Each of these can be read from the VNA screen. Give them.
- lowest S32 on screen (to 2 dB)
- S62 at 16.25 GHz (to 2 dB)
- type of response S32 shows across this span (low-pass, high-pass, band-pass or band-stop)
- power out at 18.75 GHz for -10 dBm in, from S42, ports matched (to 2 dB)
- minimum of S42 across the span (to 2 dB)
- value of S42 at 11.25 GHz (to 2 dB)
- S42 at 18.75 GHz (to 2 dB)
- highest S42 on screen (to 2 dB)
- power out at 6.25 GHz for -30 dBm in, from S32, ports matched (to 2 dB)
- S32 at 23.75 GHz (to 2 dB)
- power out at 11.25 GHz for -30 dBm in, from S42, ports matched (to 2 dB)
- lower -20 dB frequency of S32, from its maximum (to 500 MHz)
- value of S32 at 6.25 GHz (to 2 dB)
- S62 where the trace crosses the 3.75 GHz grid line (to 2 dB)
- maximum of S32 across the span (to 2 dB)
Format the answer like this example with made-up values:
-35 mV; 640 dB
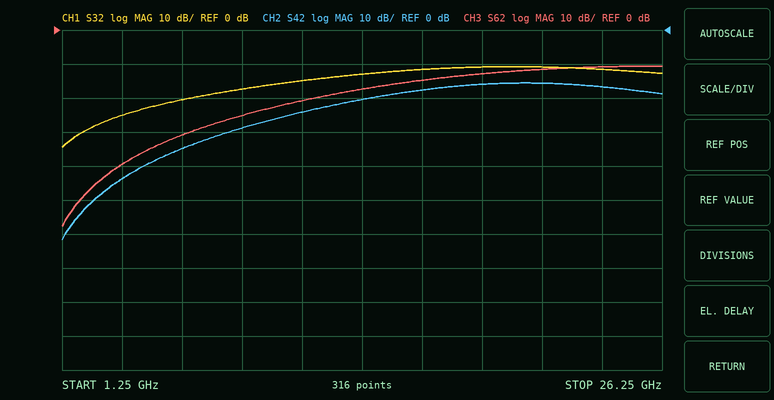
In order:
-34 dB; -14 dB; high-pass; -26 dBm; -62 dB; -24 dB; -16 dB; -16 dB; -50 dBm; -12 dB; -54 dBm; 2.0 GHz; -20 dB; -40 dB; -10 dB
